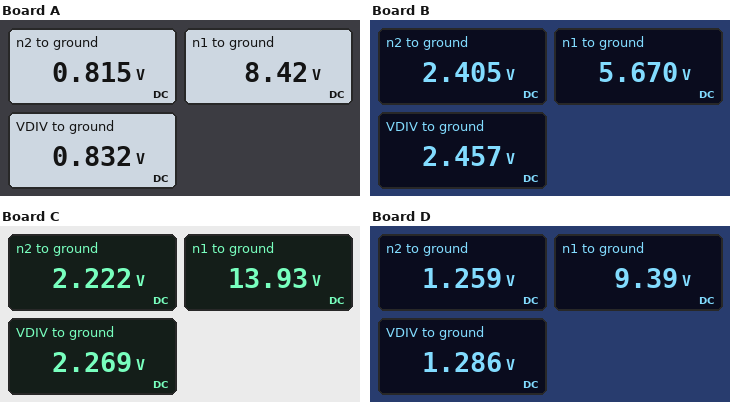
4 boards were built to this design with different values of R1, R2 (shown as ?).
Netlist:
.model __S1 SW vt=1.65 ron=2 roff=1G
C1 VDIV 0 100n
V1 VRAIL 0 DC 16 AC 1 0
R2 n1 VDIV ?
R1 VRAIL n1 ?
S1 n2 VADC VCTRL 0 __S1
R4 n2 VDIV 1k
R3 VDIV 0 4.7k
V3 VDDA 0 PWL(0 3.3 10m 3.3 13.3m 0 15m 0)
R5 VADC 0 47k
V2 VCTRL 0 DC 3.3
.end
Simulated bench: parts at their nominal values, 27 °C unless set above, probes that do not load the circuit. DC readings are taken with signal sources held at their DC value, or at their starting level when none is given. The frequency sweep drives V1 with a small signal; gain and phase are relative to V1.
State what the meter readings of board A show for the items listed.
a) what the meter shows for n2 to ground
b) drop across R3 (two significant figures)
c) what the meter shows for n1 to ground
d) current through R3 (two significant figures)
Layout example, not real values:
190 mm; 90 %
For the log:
0.815 V; 830 mV; 8.42 V; 180 µA
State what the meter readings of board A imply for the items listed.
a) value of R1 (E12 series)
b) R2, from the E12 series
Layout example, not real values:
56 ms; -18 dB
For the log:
39 kΩ; 39 kΩ
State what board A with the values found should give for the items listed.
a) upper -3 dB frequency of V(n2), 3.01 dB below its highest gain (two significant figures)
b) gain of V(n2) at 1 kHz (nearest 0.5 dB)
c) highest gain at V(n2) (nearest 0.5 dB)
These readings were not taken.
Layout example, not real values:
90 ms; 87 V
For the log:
360 Hz; -34.5 dB; -25.0 dB
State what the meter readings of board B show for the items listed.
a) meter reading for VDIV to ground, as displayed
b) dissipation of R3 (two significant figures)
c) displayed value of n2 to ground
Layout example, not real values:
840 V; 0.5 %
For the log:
2.457 V; 1.3 mW; 2.405 V
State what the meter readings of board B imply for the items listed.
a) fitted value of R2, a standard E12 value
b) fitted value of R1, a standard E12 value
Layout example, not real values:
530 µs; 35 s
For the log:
5.6 kΩ; 18 kΩ
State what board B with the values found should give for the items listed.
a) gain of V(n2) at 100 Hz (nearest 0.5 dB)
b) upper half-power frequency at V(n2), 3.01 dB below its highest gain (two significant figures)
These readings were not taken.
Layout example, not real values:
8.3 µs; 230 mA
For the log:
-16.0 dB; 410 Hz
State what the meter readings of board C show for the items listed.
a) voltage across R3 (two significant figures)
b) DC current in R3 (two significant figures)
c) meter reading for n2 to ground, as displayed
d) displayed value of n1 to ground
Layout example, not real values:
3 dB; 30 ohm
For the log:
2.3 V; 480 µA; 2.222 V; 13.93 V
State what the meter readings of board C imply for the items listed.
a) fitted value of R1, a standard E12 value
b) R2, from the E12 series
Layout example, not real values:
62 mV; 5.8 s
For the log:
3.9 kΩ; 22 kΩ
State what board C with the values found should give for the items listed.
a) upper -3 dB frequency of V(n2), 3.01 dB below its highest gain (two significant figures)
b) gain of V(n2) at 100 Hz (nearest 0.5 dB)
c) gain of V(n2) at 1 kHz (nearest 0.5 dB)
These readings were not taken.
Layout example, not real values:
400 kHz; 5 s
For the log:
400 Hz; -16.5 dB; -25.0 dB
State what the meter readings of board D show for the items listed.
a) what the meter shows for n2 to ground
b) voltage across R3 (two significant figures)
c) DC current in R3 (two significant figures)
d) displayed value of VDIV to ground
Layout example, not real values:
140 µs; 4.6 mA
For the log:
1.259 V; 1.3 V; 270 µA; 1.286 V
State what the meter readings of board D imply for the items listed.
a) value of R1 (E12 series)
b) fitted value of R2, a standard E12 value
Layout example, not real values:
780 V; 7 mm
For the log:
22 kΩ; 27 kΩ
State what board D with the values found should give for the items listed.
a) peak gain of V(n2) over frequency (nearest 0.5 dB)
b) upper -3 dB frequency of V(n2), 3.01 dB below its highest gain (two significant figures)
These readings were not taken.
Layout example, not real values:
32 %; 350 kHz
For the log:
-21.0 dB; 370 Hz
